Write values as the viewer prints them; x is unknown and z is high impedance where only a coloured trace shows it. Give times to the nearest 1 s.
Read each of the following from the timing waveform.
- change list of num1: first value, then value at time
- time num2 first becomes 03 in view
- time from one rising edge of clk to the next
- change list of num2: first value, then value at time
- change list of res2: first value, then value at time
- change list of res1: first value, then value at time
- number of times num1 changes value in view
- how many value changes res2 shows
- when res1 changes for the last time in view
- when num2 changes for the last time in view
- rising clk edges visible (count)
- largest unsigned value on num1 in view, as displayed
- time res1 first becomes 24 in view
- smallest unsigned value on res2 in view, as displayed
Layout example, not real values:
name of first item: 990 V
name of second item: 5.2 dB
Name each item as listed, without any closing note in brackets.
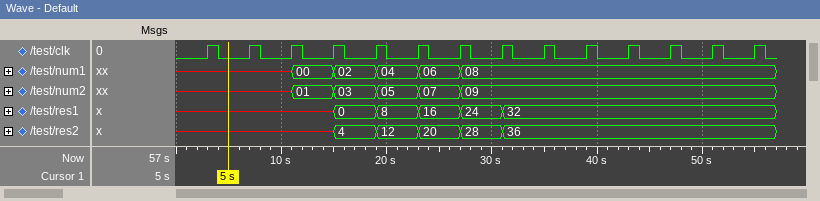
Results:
change list of num1: first value, then value at time: x, 00 at 11 s, 02 at 15 s, 04 at 19 s, 06 at 23 s, 08 at 27 s
time num2 first becomes 03 in view: 15 s
time from one rising edge of clk to the next: 4 s
change list of num2: first value, then value at time: x, 01 at 11 s, 03 at 15 s, 05 at 19 s, 07 at 23 s, 09 at 27 s
change list of res2: first value, then value at time: x, 4 at 15 s, 12 at 19 s, 20 at 23 s, 28 at 27 s, 36 at 31 s
change list of res1: first value, then value at time: x, 0 at 15 s, 8 at 19 s, 16 at 23 s, 24 at 27 s, 32 at 31 s
number of times num1 changes value in view: 5
how many value changes res2 shows: 5
when res1 changes for the last time in view: 31 s
when num2 changes for the last time in view: 27 s
rising clk edges visible: 14
largest unsigned value on num1 in view, as displayed: 08
time res1 first becomes 24 in view: 27 s
smallest unsigned value on res2 in view, as displayed: 4
